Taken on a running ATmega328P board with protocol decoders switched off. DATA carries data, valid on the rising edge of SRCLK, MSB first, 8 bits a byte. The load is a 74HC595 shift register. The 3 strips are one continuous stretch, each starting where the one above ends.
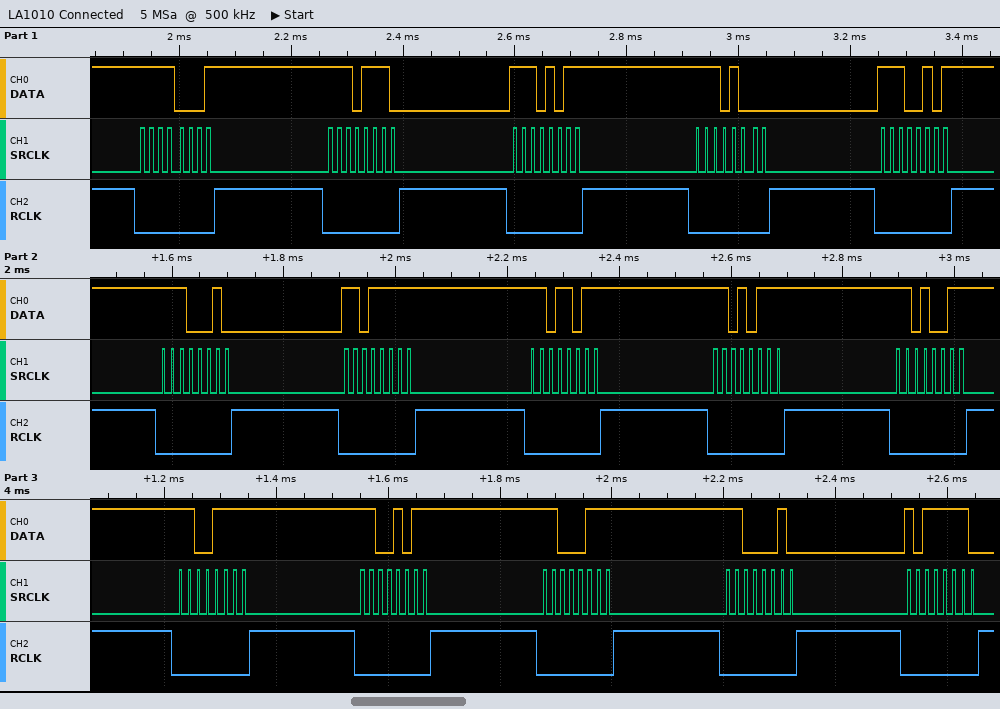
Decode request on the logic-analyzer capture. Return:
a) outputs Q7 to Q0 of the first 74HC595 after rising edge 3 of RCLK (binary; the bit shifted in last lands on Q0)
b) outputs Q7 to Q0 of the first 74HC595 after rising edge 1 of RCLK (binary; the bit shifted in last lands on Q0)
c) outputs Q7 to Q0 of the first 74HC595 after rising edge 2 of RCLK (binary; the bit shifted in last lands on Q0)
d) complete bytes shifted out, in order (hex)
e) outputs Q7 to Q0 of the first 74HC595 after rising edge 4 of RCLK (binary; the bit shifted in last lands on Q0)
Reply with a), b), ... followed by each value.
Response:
a) 11101011
b) 11110001
c) 11101110
d) F1 EE EB E8 E5 E2 DF DB D7 D3 CF CB C7 C2 BE
e) 11101000
